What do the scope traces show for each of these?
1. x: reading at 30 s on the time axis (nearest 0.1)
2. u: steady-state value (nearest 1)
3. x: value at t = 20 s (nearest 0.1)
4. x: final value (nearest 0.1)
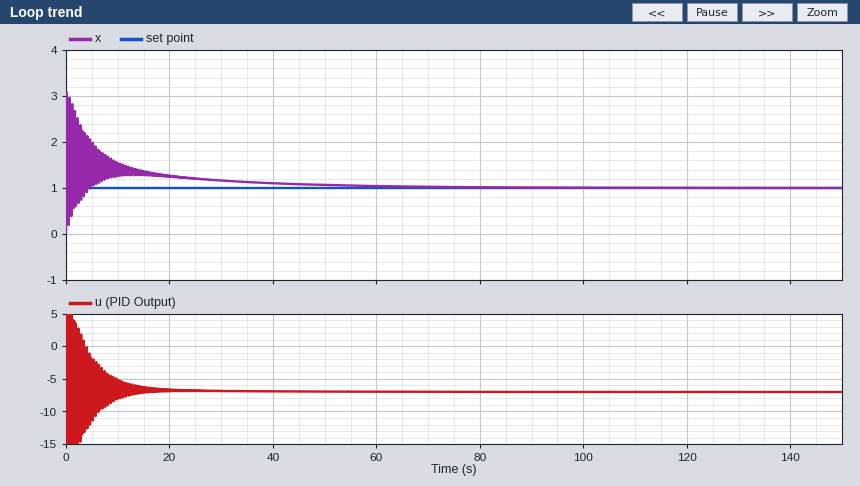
1.2
-7
1.3
1.0
